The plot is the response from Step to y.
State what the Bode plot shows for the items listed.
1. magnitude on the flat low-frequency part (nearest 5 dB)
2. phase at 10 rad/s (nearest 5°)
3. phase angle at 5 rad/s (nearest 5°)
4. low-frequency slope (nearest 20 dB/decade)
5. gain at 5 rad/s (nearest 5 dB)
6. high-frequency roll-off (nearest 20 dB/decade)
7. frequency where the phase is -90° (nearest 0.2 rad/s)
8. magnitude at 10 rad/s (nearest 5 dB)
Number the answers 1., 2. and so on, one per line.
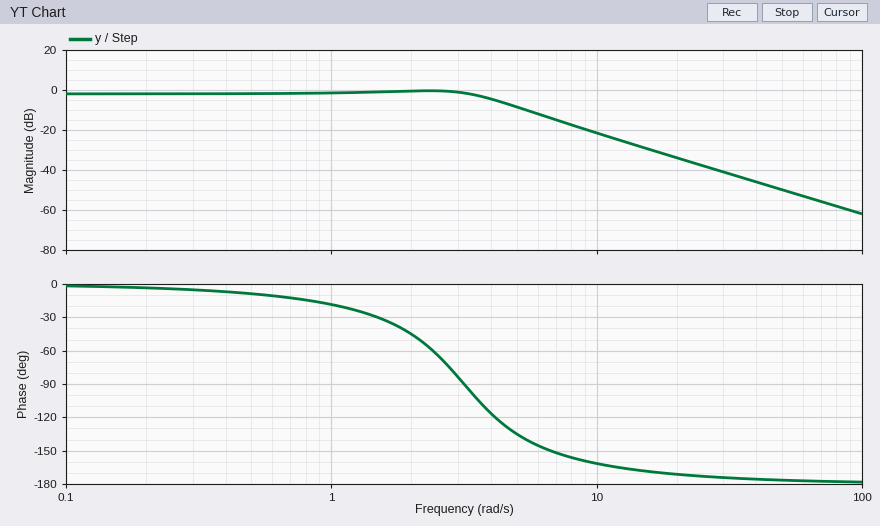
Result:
1. 0 dB
2. -160°
3. -135°
4. 0 dB/decade
5. -10 dB
6. -40 dB/decade
7. 3.2 rad/s
8. -20 dB
